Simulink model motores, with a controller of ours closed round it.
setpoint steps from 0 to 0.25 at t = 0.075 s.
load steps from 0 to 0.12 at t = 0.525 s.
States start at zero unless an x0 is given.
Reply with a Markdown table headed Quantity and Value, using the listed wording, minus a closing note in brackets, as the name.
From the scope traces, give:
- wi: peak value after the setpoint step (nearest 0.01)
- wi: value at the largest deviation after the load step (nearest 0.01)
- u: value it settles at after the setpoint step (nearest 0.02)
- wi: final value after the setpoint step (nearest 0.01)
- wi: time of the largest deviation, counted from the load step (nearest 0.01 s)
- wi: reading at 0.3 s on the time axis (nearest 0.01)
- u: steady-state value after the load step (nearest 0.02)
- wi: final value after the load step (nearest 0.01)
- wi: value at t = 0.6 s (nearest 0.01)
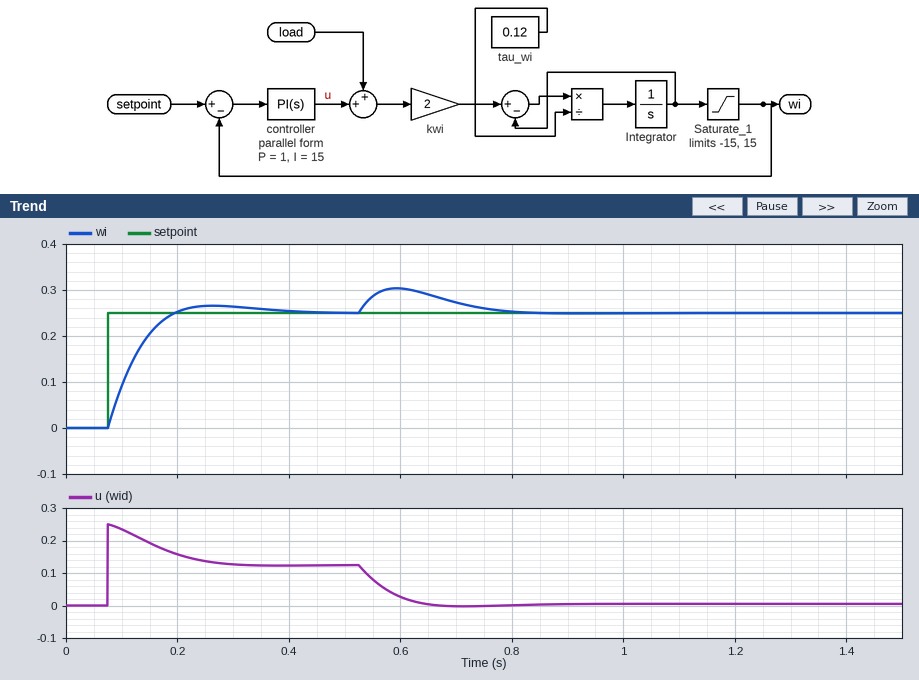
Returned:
| Quantity | Value |
|---|---|
| wi: peak value after the setpoint step | 0.27 |
| wi: value at the largest deviation after the load step | 0.30 |
| u: value it settles at after the setpoint step | 0.12 |
| wi: final value after the setpoint step | 0.25 |
| wi: time of the largest deviation, counted from the load step | 0.07 s |
| wi: reading at 0.3 s on the time axis | 0.26 |
| u: steady-state value after the load step | 0.00 |
| wi: final value after the load step | 0.25 |
| wi: value at t = 0.6 s | 0.30 |
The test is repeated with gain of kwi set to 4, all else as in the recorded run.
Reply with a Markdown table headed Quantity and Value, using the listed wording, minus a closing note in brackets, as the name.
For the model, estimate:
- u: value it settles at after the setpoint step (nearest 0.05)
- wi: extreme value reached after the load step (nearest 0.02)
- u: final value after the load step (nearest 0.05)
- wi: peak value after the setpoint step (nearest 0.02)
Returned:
| Quantity | Value |
|---|---|
| u: value it settles at after the setpoint step | 0.05 |
| wi: extreme value reached after the load step | 0.32 |
| u: final value after the load step | -0.05 |
| wi: peak value after the setpoint step | 0.26 |
